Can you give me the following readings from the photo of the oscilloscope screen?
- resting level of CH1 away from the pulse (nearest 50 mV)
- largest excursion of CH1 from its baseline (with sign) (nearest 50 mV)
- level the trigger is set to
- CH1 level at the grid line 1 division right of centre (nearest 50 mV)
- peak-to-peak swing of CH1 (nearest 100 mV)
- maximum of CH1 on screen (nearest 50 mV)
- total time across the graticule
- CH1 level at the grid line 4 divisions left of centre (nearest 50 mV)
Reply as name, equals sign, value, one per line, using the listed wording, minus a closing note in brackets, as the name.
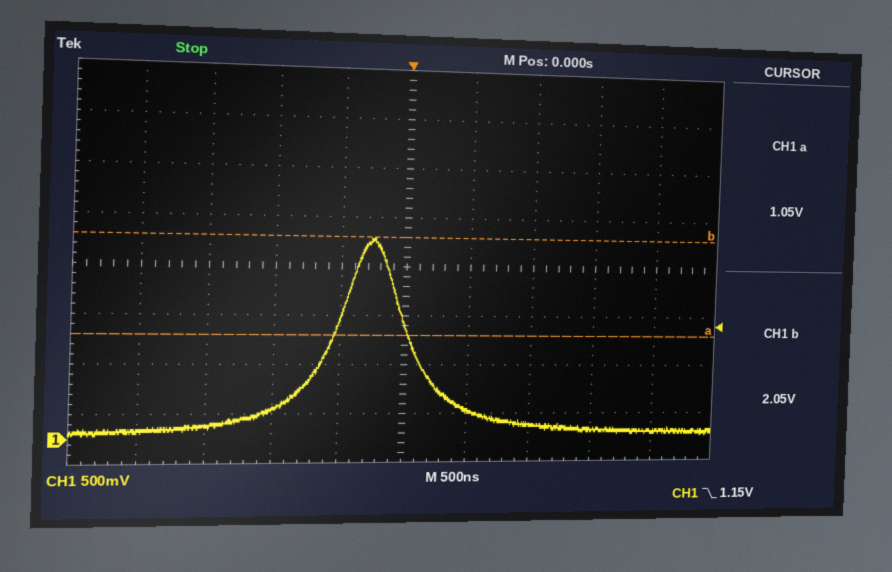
resting level of CH1 away from the pulse = 100 mV
largest excursion of CH1 from its baseline (with sign) = +1.95 V
level the trigger is set to = 1.15 V
CH1 level at the grid line 1 division right of centre = 300 mV
peak-to-peak swing of CH1 = 2.00 V
maximum of CH1 on screen = 2.05 V
total time across the graticule = 5 µs
CH1 level at the grid line 4 divisions left of centre = 100 mV
